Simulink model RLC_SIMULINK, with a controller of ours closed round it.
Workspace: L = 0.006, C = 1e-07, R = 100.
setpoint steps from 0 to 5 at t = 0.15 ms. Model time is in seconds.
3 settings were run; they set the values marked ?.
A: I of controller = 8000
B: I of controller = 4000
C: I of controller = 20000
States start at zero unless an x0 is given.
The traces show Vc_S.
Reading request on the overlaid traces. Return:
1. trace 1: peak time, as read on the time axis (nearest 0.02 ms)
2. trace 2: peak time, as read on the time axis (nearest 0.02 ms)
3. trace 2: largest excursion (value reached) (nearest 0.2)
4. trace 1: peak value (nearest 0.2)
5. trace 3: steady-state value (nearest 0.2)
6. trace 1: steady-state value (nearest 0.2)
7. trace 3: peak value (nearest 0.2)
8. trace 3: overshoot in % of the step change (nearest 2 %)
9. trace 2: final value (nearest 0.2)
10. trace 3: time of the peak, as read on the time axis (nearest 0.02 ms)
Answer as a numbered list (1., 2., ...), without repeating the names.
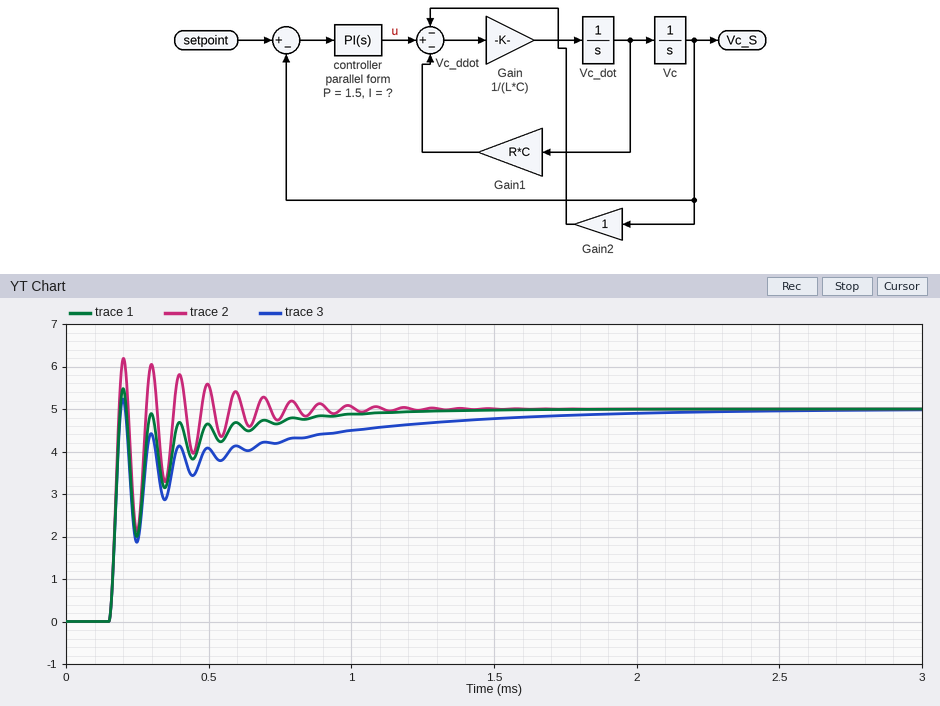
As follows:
1. 0.20 ms
2. 0.20 ms
3. 6.2
4. 5.4
5. 5.0
6. 5.0
7. 5.2
8. 4 %
9. 5.0
10. 0.20 ms
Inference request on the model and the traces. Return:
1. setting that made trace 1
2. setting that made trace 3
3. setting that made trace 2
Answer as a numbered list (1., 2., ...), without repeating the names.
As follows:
1. A
2. B
3. C
